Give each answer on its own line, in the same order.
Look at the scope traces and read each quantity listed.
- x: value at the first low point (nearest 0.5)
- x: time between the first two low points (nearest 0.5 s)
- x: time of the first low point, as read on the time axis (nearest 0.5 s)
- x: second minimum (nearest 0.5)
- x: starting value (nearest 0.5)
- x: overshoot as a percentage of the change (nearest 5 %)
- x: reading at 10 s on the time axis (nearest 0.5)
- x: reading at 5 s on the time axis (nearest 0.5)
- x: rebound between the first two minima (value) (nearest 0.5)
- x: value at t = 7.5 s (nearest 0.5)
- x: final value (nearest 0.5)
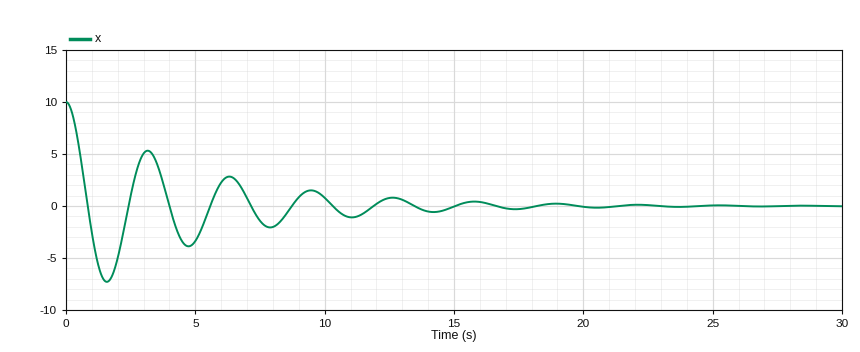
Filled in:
-7.5
3.0 s
1.5 s
-4.0
10.0
75 %
1.0
-3.5
5.5
-1.5
0.0
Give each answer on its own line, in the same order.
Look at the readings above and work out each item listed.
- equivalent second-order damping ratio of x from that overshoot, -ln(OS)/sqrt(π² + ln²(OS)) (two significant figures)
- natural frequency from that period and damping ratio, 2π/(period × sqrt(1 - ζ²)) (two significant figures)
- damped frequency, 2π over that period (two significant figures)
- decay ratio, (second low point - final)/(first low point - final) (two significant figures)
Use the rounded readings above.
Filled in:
0.091
2.1 rad/s
2.1 rad/s
0.53
